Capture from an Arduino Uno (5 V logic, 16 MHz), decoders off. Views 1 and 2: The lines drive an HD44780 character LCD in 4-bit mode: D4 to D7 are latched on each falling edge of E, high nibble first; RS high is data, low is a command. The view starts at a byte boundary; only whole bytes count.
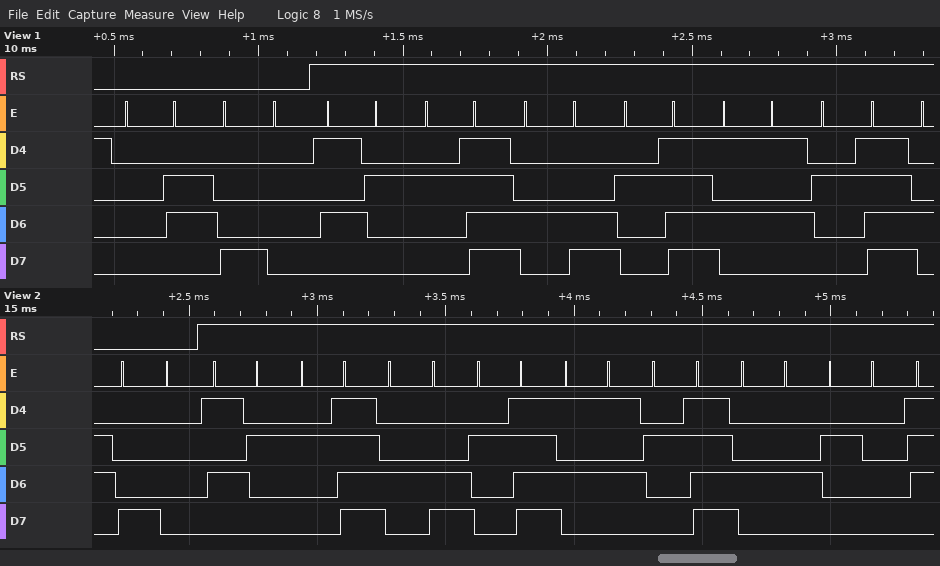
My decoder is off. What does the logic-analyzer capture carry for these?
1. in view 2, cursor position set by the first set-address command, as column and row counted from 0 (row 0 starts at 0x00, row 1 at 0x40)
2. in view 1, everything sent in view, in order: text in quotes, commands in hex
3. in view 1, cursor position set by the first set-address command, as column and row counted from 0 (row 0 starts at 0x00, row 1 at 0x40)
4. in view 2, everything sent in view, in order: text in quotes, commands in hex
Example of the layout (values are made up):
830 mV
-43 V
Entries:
column 0, row 0
0x06 0x80 "R/L/U/"
column 0, row 0
0x80 "R/L/U/D "
